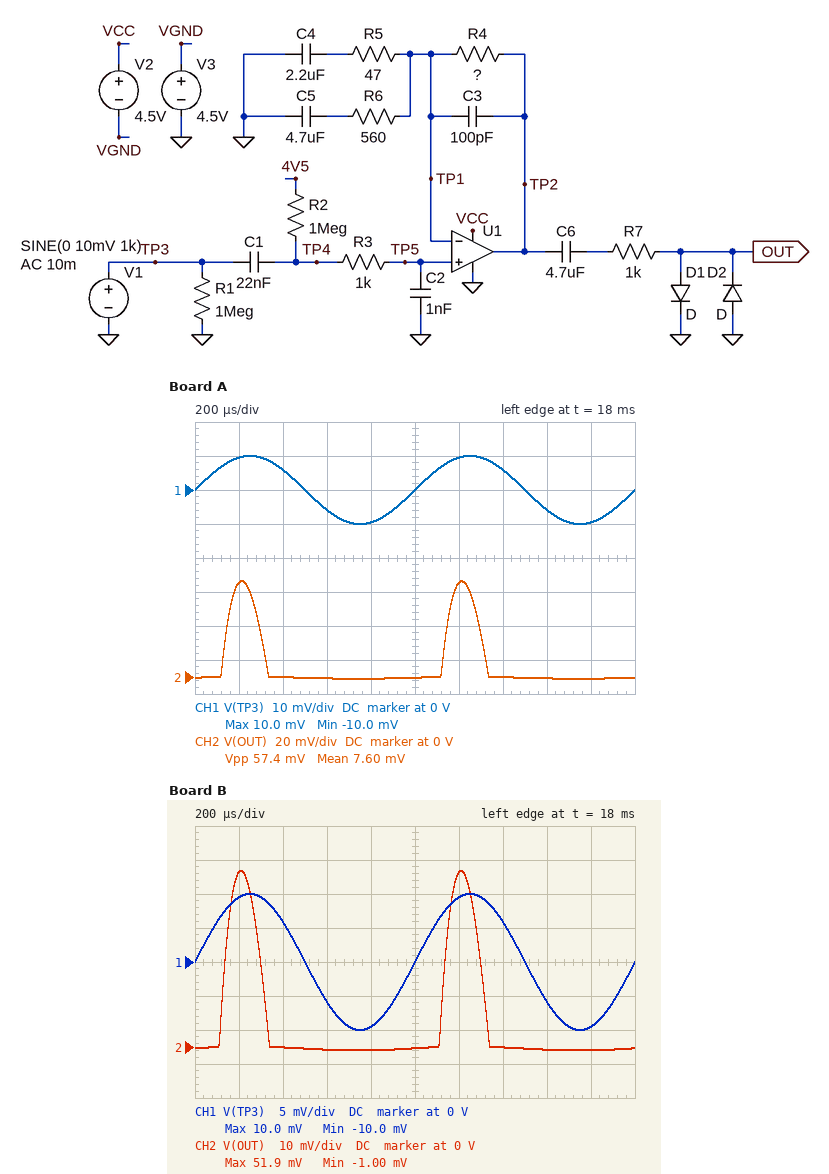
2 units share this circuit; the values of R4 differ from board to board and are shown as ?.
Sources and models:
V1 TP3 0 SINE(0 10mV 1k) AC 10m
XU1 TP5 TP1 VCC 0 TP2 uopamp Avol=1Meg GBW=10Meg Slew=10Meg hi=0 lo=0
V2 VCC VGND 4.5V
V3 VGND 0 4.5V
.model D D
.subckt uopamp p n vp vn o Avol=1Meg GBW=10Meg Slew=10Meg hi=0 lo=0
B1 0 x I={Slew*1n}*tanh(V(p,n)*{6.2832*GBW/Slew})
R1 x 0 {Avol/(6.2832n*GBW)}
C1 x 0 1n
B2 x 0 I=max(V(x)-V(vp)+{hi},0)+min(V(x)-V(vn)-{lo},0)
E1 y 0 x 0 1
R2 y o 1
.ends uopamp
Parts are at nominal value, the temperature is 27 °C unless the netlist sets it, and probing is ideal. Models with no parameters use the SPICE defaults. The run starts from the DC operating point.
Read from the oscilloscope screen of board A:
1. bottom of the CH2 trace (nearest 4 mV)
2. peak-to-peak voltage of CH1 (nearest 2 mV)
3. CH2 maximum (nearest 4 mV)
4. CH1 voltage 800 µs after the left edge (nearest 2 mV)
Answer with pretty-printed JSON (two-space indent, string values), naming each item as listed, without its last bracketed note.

{
  "bottom of the CH2 trace": "0 V",
  "peak-to-peak voltage of CH1": "20 mV",
  "CH2 maximum": "56 mV",
  "CH1 voltage 800 µs after the left edge": "-10 mV"
}
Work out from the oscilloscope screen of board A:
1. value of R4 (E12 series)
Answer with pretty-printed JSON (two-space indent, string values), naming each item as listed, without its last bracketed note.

{
  "value of R4": "1.2 kΩ"
}
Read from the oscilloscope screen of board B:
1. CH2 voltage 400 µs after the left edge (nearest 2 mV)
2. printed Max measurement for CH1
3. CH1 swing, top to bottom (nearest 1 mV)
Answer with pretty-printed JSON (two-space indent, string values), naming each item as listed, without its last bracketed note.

{
  "CH2 voltage 400 µs after the left edge": "0 V",
  "printed Max measurement for CH1": "10.0 mV",
  "CH1 swing, top to bottom": "20 mV"
}
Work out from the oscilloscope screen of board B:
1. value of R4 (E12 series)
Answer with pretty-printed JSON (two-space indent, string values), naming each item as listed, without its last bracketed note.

{
  "value of R4": "1 kΩ"
}
